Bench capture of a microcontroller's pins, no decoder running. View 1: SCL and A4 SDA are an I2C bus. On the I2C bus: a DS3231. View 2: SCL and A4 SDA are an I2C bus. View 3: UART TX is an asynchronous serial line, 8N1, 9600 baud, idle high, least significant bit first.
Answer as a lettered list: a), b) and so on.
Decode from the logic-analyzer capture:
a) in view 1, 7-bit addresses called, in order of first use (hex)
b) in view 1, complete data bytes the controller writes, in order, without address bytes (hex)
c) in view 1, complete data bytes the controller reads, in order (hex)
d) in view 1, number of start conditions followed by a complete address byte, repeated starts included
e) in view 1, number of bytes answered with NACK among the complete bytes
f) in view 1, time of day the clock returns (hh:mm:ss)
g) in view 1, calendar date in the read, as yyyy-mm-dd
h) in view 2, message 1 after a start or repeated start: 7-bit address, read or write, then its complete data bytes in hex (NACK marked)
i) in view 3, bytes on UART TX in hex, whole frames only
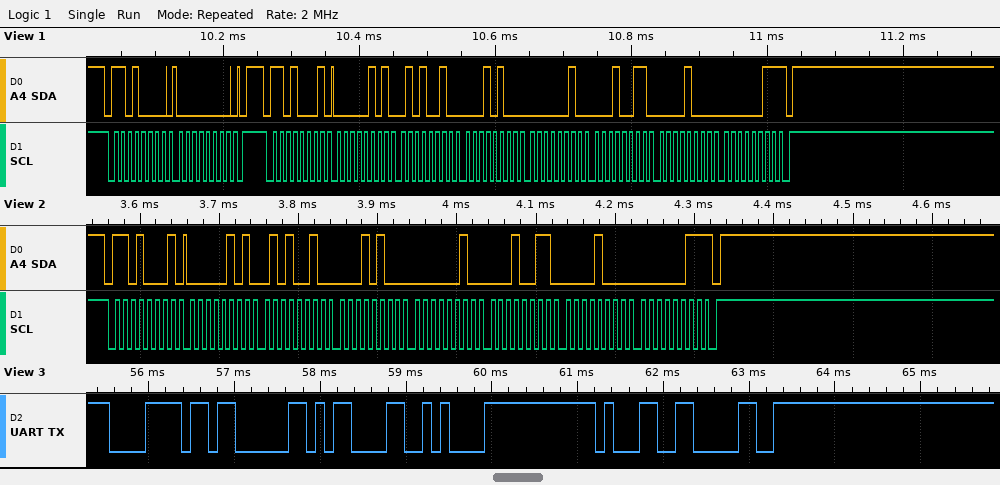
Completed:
a) 0x68
b) 00
c) 05 52 14 02 13 08 03
d) 2
e) 1
f) 14:52:05
g) 2003-08-13
h) 0x68 read: 05 52 14 02 13 08 03 NACK
i) 0x78 0x03 0x0D 0x0A 0x31 0x30
